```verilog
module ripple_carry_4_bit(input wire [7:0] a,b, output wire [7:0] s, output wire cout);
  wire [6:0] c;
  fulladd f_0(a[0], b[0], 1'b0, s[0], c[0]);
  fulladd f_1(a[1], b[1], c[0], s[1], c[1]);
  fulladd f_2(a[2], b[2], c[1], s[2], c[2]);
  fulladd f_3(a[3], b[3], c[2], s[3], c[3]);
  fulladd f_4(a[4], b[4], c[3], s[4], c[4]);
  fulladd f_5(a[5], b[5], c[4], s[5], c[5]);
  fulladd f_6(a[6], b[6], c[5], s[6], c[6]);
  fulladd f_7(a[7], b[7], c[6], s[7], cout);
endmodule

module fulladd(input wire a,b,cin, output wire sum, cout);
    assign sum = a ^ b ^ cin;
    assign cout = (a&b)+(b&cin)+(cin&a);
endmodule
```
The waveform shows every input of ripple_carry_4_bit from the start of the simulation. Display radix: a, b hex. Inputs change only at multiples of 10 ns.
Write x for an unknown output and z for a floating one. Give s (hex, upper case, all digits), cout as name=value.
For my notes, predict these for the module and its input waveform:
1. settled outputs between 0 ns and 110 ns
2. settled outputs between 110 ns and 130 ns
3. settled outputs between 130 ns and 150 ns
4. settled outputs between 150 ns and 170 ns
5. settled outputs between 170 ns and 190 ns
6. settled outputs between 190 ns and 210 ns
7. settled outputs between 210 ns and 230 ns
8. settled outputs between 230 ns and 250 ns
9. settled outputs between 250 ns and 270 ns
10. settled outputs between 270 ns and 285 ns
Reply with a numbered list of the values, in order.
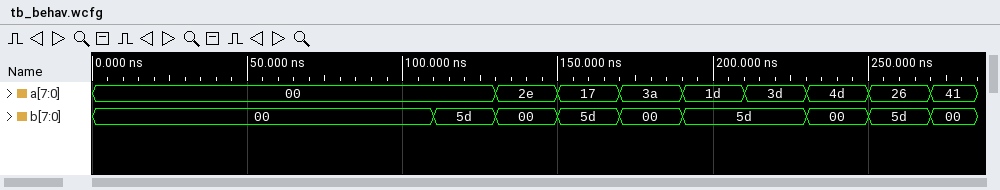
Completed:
1. s=00, cout=0
2. s=5D, cout=0
3. s=2E, cout=0
4. s=74, cout=0
5. s=3A, cout=0
6. s=7A, cout=0
7. s=9A, cout=0
8. s=4D, cout=0
9. s=83, cout=0
10. s=41, cout=0
